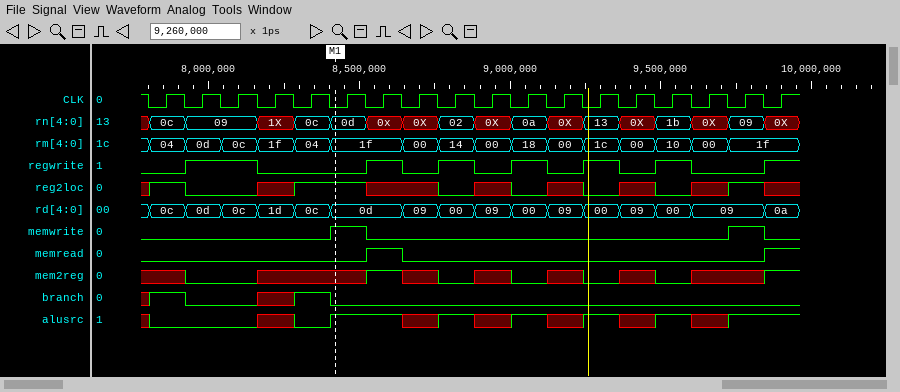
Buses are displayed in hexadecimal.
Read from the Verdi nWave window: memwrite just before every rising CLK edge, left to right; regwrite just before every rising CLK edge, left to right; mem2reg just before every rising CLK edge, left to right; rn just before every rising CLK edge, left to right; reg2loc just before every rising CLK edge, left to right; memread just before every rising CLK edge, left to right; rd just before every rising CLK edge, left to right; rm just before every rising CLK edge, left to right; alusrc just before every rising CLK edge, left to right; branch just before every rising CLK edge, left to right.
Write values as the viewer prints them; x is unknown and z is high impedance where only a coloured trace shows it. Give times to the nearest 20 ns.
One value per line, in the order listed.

0 0 0 0 0 1 0 0 0 0 0 0 0 0 0 0 1 0
0 1 1 0 0 0 1 0 1 0 1 0 1 0 1 0 0 1
x 0 0 x x x 1 x 0 x 0 x 0 x 0 x x 1
0c, 09, 09, 1X, 0c, 0d, 0x, 0X, 02, 0X, 0a, 0X, 13, 0X, 1b, 0X, 09, 0X
1 0 0 x 1 1 x x 0 x 0 x 0 x 0 x 1 x
0 0 0 0 0 0 1 0 0 0 0 0 0 0 0 0 0 1
0c, 0d, 0c, 1d, 0c, 0d, 0d, 09, 00, 09, 00, 09, 00, 09, 00, 09, 09, 0a
04, 0d, 0c, 1f, 04, 1f, 1f, 00, 14, 00, 18, 00, 1c, 00, 10, 00, 1f, 1f
0 0 0 x 0 1 1 x 1 x 1 x 1 x 1 x 1 1
1 0 0 x 1 0 0 0 0 0 0 0 0 0 0 0 0 0
